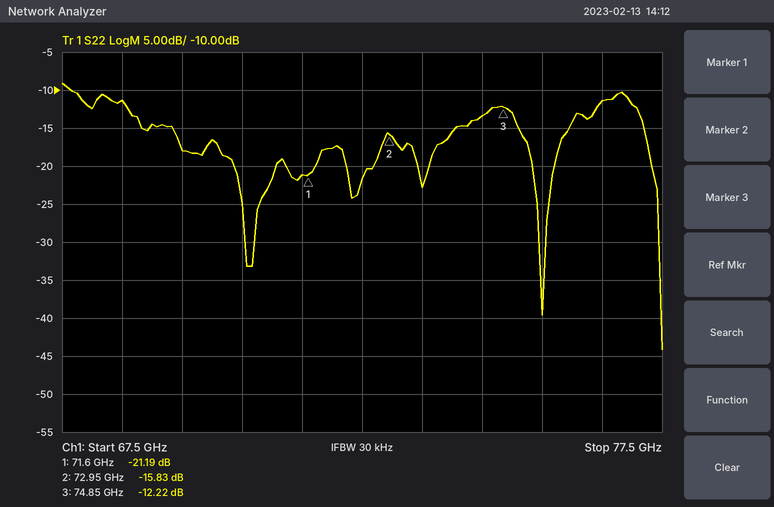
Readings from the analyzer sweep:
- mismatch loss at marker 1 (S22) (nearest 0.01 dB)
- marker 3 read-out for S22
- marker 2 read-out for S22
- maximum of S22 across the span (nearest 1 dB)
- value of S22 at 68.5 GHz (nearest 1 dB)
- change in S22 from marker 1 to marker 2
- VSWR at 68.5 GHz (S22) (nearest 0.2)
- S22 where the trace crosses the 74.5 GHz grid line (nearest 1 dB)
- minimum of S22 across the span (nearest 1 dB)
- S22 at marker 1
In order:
0.03 dB
-12.22 dB
-15.83 dB
-9 dB
-11 dB
5.36 dB
1.8
-13 dB
-44 dB
-21.19 dB
